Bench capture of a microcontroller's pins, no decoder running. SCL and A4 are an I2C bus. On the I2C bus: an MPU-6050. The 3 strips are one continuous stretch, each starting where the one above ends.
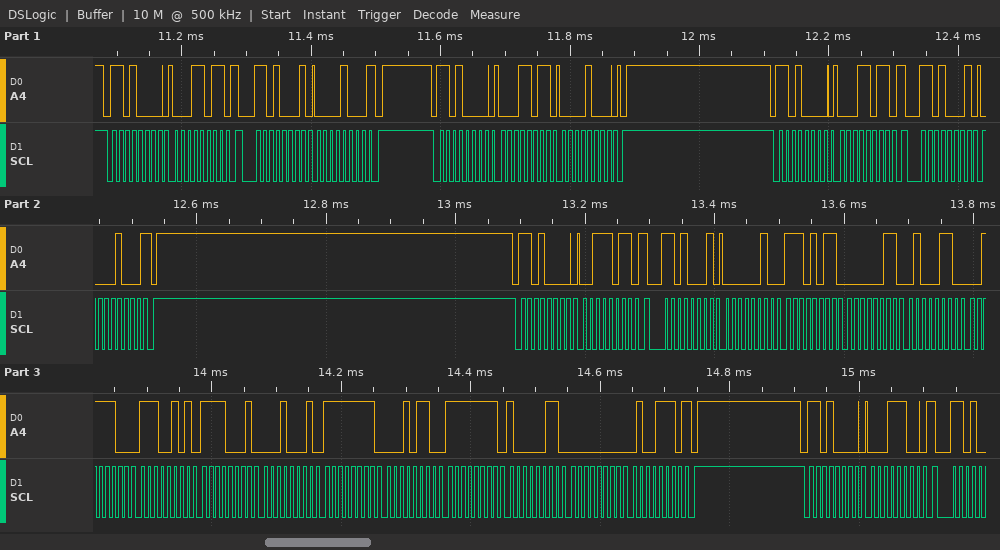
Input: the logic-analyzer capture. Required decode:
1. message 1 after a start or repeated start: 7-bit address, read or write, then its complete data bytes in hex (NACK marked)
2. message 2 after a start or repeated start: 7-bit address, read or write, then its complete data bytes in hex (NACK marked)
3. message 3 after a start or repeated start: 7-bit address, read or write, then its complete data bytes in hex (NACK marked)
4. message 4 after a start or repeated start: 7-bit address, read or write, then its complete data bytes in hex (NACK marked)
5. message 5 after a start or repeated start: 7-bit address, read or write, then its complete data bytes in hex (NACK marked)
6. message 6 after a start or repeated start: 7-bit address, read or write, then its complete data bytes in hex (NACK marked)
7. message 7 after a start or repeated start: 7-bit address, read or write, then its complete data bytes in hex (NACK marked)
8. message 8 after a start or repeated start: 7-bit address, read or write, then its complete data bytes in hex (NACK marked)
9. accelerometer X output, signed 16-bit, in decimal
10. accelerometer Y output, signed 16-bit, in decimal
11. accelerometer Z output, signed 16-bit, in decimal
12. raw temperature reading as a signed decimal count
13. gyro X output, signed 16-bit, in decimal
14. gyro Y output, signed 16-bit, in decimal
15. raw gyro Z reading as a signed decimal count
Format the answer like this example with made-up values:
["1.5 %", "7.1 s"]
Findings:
["0x68 write: 1B", "0x68 read: 08 NACK", "0x68 write: 1B 08", "0x68 write: 1B", "0x68 read: 08 NACK", "0x68 write: 3B", "0x68 read: 02 EB 03 46 3C E5 F1 11 FF 16 FF 83 00 4E NACK", "0x68 write: 1C", "747", "838", "15589", "-3823", "-234", "-125", "78"]
